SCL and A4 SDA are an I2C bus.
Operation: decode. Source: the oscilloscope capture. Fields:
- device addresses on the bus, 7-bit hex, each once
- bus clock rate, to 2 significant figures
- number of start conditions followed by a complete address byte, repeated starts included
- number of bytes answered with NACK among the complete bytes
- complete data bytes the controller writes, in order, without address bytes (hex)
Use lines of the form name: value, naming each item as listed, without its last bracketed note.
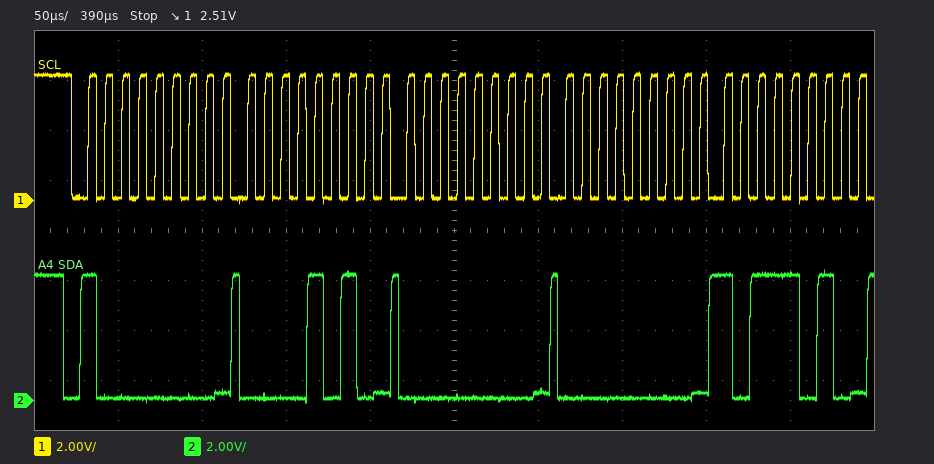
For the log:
device addresses on the bus, 7-bit hex, each once: 0x40
bus clock rate, to 2 significant figures: 100 kHz
number of start conditions followed by a complete address byte, repeated starts included: 1
number of bytes answered with NACK among the complete bytes: 0
complete data bytes the controller writes, in order, without address bytes: 0A 00 00 BA
